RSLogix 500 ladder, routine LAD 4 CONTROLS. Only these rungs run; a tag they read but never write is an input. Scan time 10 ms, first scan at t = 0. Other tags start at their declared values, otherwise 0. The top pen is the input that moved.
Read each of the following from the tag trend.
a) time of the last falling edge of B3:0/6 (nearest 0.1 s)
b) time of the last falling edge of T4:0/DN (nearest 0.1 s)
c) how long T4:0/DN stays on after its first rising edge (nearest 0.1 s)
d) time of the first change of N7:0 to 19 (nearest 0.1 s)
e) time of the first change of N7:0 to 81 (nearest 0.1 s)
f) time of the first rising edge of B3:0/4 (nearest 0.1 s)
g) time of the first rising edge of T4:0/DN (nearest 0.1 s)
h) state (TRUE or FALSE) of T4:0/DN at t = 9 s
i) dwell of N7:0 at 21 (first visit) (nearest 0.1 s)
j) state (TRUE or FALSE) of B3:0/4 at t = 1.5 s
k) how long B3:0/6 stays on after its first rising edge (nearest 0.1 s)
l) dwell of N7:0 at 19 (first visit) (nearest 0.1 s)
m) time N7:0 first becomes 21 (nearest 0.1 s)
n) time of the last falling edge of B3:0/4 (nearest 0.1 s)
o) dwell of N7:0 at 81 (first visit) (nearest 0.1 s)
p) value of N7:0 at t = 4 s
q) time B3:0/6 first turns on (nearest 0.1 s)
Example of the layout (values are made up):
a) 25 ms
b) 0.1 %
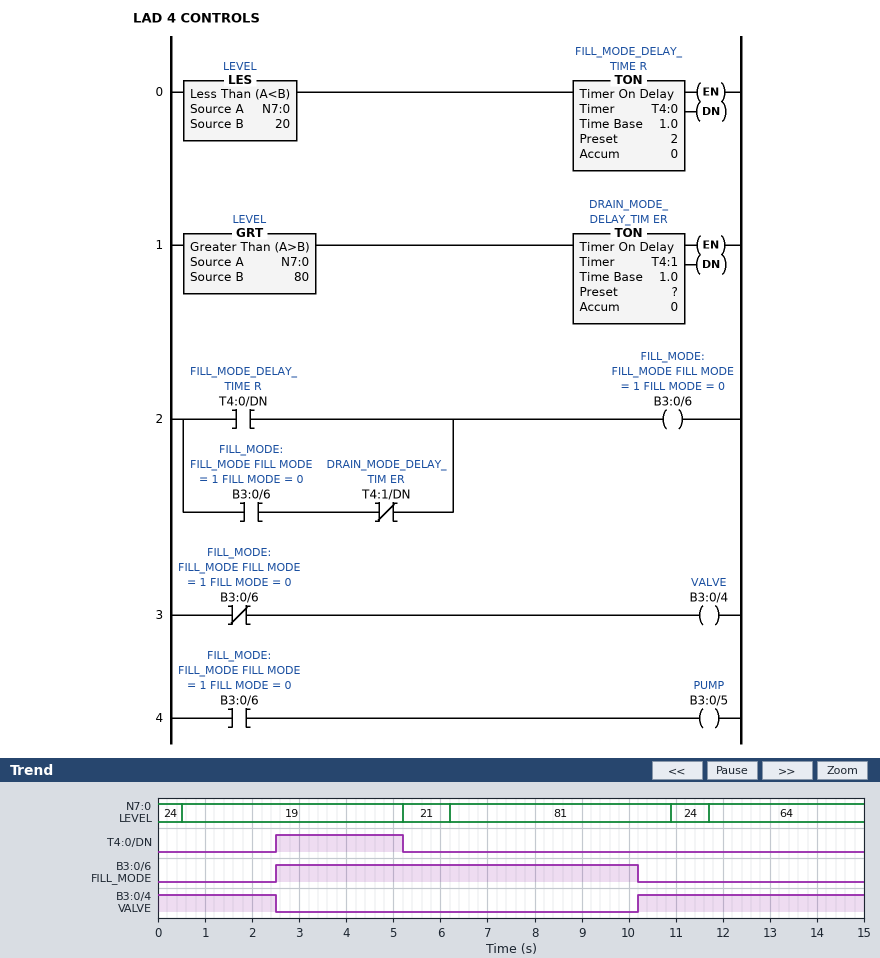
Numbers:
a) 10.2 s
b) 5.2 s
c) 2.7 s
d) 0.5 s
e) 6.2 s
f) 10.2 s
g) 2.5 s
h) FALSE
i) 1.0 s
j) TRUE
k) 7.7 s
l) 4.7 s
m) 5.2 s
n) 2.5 s
o) 4.7 s
p) 19
q) 2.5 s
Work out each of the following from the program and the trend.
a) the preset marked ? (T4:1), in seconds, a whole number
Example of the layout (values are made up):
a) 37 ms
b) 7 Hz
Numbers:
a) 4 s
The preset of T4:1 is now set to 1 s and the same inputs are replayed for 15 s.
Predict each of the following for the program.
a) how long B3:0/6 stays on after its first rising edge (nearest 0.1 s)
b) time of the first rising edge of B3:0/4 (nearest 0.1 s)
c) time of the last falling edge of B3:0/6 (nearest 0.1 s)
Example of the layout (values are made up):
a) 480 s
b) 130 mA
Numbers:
a) 4.7 s
b) 7.2 s
c) 7.2 s
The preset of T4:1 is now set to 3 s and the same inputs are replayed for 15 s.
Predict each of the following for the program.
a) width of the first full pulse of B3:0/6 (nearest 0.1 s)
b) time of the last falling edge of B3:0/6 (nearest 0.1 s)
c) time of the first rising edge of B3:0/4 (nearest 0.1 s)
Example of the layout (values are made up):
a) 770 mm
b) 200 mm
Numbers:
a) 6.7 s
b) 9.2 s
c) 9.2 s
